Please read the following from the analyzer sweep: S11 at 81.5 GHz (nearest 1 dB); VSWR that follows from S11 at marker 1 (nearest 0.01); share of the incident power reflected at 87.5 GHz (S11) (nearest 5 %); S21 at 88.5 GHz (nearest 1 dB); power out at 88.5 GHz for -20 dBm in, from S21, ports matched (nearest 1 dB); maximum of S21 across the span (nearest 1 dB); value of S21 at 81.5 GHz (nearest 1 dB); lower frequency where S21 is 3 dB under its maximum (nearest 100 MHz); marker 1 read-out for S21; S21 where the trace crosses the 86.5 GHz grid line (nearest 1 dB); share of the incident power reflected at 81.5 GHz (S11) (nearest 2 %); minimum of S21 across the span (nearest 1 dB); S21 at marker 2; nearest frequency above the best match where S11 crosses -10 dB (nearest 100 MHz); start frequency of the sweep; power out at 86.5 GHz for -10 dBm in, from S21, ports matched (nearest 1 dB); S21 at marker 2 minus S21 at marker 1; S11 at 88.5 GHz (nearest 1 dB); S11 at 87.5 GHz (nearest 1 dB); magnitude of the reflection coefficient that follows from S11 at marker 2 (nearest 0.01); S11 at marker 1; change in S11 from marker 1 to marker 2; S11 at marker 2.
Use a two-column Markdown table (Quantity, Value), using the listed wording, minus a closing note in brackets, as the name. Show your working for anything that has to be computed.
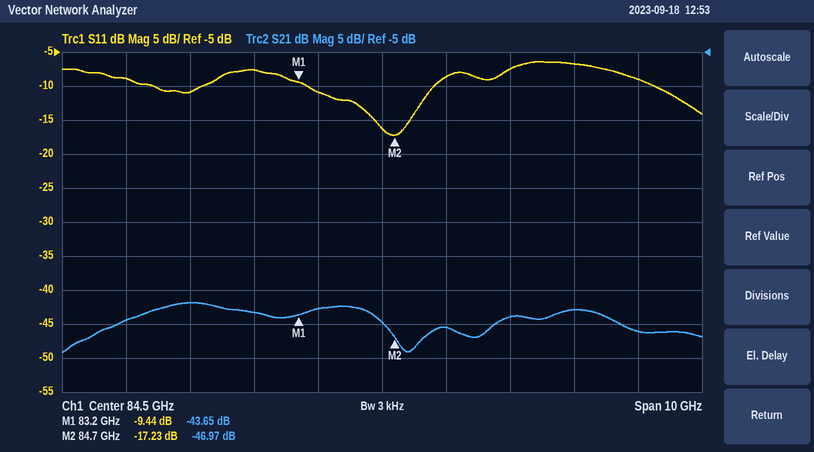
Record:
| Quantity | Value |
|---|---|
| S11 at 81.5 GHz | -11 dB |
| VSWR that follows from S11 at marker 1 | (1 + 0.3373)/(1 − 0.3373) ≈ 2.02 |
| share of the incident power reflected at 87.5 GHz (S11) | 10^(-7/10) ≈ 20 % |
| S21 at 88.5 GHz | -46 dB |
| power out at 88.5 GHz for -20 dBm in, from S21, ports matched | -20 dBm + (-46 dB) = -66 dBm |
| maximum of S21 across the span | -42 dB |
| value of S21 at 81.5 GHz | -42 dB |
| lower frequency where S21 is 3 dB under its maximum | 80.4 GHz |
| marker 1 read-out for S21 | -43.65 dB |
| S21 where the trace crosses the 86.5 GHz grid line | -44 dB |
| share of the incident power reflected at 81.5 GHz (S11) | 10^(-11/10) ≈ 8 % |
| minimum of S21 across the span | -49 dB |
| S21 at marker 2 | -46.97 dB |
| nearest frequency above the best match where S11 crosses -10 dB | 85.3 GHz |
| start frequency of the sweep | 79.5 GHz |
| power out at 86.5 GHz for -10 dBm in, from S21, ports matched | -10 dBm + (-44 dB) = -54 dBm |
| S21 at marker 2 minus S21 at marker 1 | -46.97 − (-43.65) = -3.32 dB |
| S11 at 88.5 GHz | -9 dB |
| S11 at 87.5 GHz | -7 dB |
| magnitude of the reflection coefficient that follows from S11 at marker 2 | 10^(-17.23/20) ≈ 0.14 |
| S11 at marker 1 | -9.44 dB |
| change in S11 from marker 1 to marker 2 | -17.23 − (-9.44) = -7.79 dB |
| S11 at marker 2 | -17.23 dB |
